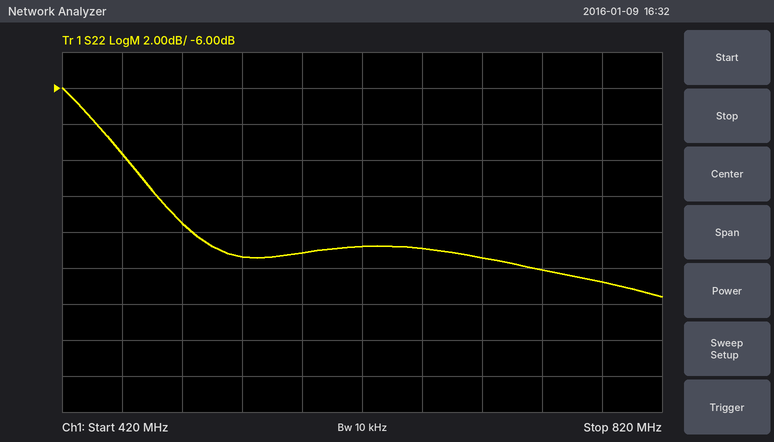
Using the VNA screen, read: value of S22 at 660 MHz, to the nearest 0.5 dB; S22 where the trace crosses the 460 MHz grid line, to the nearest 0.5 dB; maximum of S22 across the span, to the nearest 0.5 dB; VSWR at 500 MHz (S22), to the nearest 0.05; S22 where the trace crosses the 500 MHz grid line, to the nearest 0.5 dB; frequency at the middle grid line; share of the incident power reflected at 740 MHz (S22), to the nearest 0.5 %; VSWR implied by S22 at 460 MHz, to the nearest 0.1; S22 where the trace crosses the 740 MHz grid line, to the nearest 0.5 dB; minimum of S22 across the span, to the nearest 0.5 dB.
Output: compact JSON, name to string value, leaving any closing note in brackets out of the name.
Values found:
{"value of S22 at 660 MHz, to the nearest 0.5 dB": "-15.0 dB", "S22 where the trace crosses the 460 MHz grid line, to the nearest 0.5 dB": "-9.5 dB", "maximum of S22 across the span, to the nearest 0.5 dB": "-6.0 dB", "VSWR at 500 MHz (S22), to the nearest 0.05": "1.55", "S22 where the trace crosses the 500 MHz grid line, to the nearest 0.5 dB": "-13.5 dB", "frequency at the middle grid line": "620 MHz", "share of the incident power reflected at 740 MHz (S22), to the nearest 0.5 %": "2.5 %", "VSWR implied by S22 at 460 MHz, to the nearest 0.1": "2.0", "S22 where the trace crosses the 740 MHz grid line, to the nearest 0.5 dB": "-16.0 dB", "minimum of S22 across the span, to the nearest 0.5 dB": "-17.5 dB"}
